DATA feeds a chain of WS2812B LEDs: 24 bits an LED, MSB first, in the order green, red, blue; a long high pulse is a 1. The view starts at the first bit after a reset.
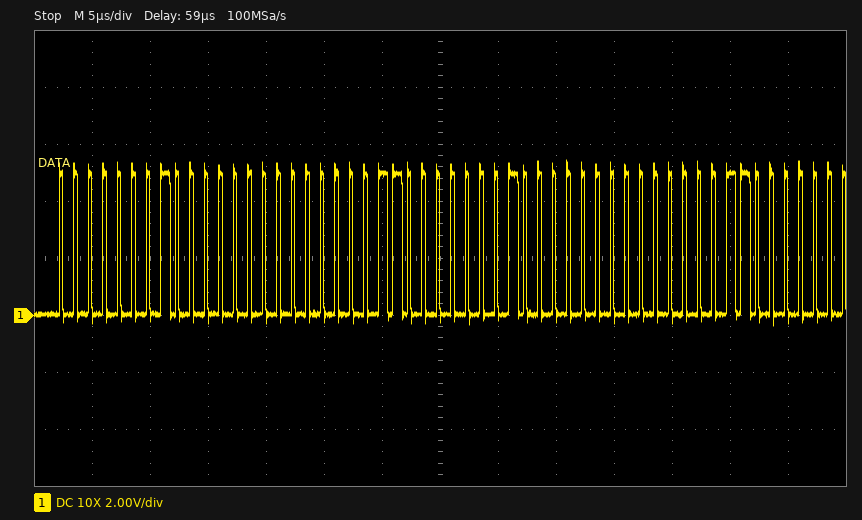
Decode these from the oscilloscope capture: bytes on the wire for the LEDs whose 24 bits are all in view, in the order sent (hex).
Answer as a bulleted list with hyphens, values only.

- 01 00 03 01 00 03
